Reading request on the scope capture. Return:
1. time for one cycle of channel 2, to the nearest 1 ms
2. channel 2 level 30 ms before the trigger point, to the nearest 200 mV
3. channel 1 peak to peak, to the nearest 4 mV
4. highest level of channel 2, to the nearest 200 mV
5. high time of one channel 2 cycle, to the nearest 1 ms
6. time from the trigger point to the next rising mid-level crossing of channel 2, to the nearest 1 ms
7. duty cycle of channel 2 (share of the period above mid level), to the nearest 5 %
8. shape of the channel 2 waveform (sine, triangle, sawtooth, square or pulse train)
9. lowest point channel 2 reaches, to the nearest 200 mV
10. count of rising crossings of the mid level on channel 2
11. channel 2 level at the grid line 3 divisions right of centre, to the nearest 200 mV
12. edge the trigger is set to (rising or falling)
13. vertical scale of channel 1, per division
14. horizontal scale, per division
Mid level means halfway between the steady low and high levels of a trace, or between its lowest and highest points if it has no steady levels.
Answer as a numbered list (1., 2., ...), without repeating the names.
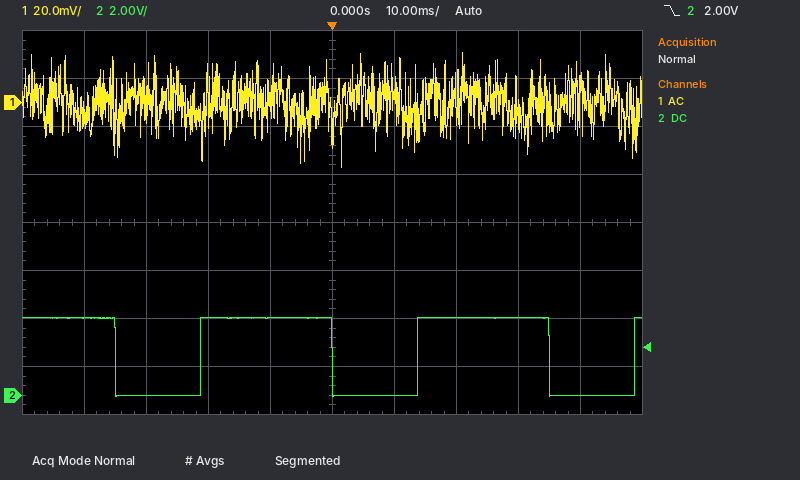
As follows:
1. 35 ms
2. 0.0 V
3. 48 mV
4. 3.2 V
5. 21 ms
6. 14 ms
7. 60 %
8. pulse train
9. 0.0 V
10. 3
11. 3.2 V
12. falling
13. 20 mV
14. 10 ms
